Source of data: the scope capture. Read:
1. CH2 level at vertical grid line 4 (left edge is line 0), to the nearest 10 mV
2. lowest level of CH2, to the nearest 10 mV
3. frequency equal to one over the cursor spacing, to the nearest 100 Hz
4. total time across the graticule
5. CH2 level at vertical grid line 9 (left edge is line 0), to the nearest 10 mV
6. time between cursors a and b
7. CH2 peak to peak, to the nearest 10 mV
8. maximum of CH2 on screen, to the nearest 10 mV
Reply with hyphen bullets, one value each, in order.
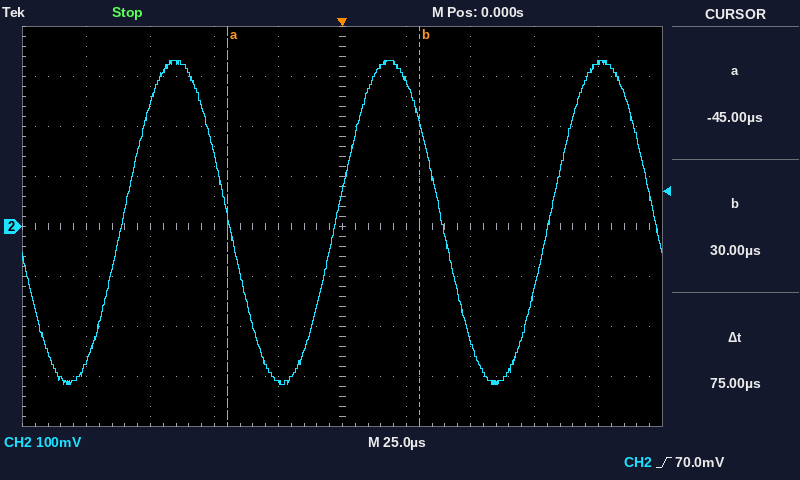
- -310 mV
- -320 mV
- 13.3 kHz
- 250 µs
- 330 mV
- 75 µs
- 650 mV
- 330 mV
